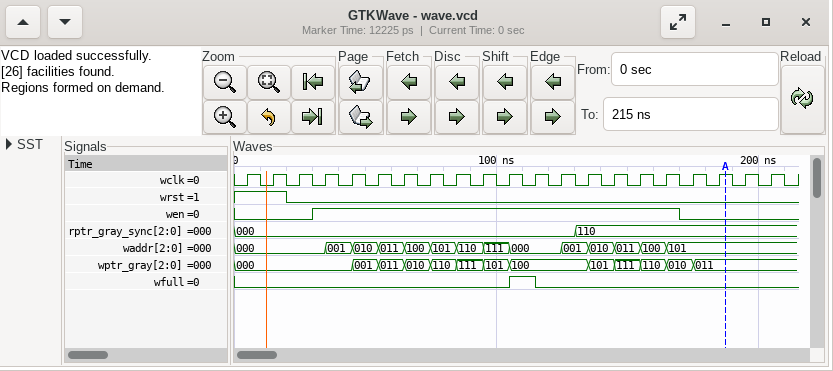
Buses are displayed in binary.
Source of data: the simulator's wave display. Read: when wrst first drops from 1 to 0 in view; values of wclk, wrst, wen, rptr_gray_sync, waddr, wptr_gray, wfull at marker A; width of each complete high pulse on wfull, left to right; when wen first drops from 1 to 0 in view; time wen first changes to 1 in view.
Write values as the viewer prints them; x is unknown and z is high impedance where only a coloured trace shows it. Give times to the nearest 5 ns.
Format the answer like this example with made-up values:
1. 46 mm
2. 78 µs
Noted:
1. 20 ns
2. wclk=1, wrst=0, wen=0, rptr_gray_sync=110, waddr=101, wptr_gray=011, wfull=0
3. 10 ns
4. 170 ns
5. 30 ns
